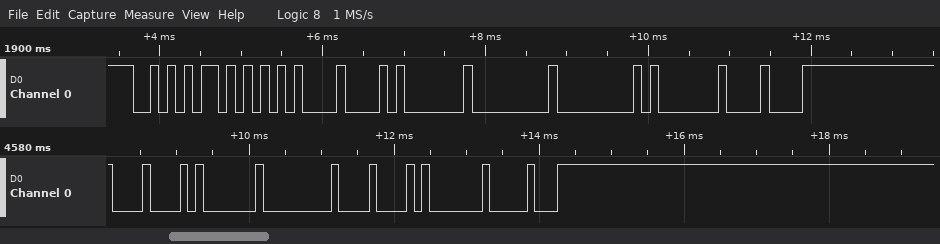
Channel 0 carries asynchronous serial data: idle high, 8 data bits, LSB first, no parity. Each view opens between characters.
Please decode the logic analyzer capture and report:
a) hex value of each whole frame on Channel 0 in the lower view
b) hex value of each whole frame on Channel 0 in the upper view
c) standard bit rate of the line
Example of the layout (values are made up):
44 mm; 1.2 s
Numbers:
08, 01, 00, 08, 01, 10; AA, 55, 08, 01, 00, 00, 01, 08; 9600 baud
